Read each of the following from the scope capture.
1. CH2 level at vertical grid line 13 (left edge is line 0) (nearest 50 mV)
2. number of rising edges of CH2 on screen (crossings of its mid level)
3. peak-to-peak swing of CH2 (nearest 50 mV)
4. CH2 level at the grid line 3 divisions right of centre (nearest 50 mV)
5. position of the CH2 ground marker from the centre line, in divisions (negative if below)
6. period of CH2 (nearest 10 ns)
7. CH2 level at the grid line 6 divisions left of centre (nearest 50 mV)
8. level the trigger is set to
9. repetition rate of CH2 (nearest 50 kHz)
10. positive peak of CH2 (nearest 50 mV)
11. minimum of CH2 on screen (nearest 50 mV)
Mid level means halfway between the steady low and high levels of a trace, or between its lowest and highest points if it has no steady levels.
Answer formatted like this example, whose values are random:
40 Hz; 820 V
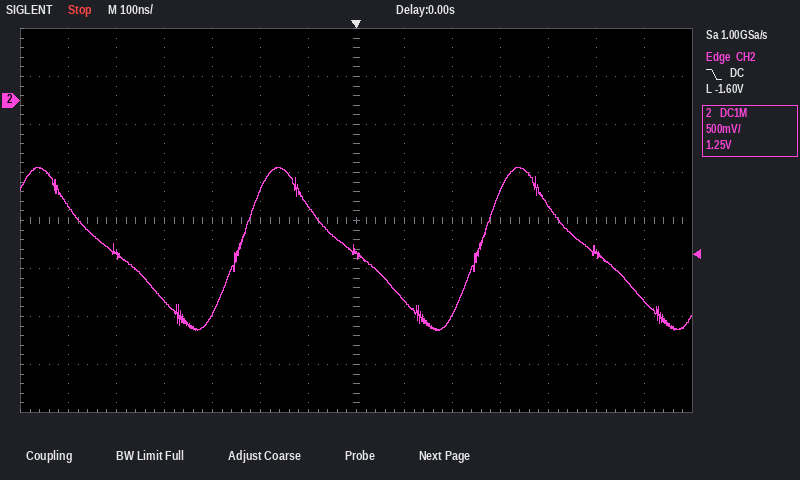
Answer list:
-2.10 V; 2; 1.70 V; -950 mV; +2.5 div; 500 ns; -1.10 V; -1.60 V; 2.00 MHz; -700 mV; -2.40 V
